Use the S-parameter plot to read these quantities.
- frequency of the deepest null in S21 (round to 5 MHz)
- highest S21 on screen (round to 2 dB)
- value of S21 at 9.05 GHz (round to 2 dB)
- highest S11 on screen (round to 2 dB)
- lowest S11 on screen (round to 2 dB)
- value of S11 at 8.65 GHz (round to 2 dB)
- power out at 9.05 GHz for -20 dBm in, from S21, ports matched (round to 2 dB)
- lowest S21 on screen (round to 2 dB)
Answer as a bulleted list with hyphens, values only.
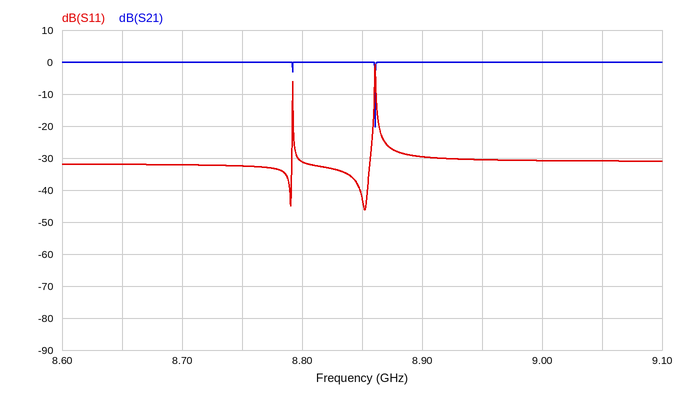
- 8.860 GHz
- 0 dB
- 0 dB
- 0 dB
- -46 dB
- -32 dB
- -20 dBm
- -20 dB
